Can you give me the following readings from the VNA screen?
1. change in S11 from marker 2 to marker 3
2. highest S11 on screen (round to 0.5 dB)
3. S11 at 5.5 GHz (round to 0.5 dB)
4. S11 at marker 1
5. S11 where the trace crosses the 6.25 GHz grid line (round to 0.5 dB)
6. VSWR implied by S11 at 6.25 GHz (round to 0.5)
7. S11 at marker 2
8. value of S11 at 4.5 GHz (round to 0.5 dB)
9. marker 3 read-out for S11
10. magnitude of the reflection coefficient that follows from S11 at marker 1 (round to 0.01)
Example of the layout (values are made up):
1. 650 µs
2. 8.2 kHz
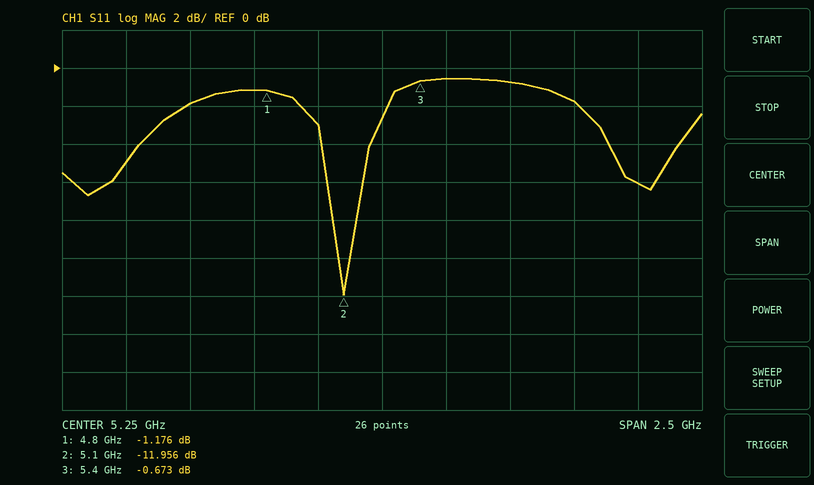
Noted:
1. 11.283 dB
2. -0.5 dB
3. -0.5 dB
4. -1.176 dB
5. -6.0 dB
6. 3.0
7. -11.956 dB
8. -2.0 dB
9. -0.673 dB
10. 0.87
